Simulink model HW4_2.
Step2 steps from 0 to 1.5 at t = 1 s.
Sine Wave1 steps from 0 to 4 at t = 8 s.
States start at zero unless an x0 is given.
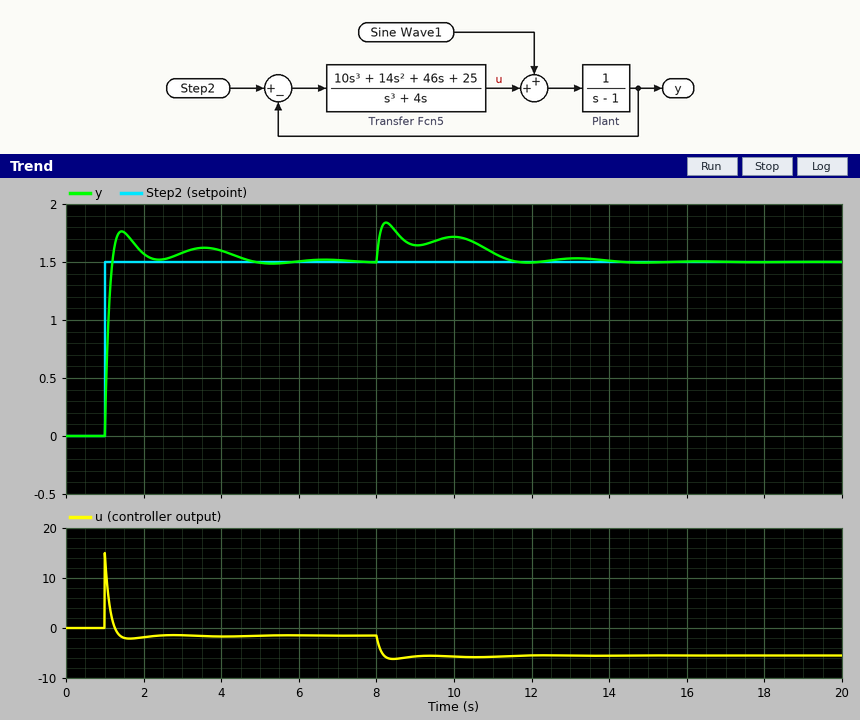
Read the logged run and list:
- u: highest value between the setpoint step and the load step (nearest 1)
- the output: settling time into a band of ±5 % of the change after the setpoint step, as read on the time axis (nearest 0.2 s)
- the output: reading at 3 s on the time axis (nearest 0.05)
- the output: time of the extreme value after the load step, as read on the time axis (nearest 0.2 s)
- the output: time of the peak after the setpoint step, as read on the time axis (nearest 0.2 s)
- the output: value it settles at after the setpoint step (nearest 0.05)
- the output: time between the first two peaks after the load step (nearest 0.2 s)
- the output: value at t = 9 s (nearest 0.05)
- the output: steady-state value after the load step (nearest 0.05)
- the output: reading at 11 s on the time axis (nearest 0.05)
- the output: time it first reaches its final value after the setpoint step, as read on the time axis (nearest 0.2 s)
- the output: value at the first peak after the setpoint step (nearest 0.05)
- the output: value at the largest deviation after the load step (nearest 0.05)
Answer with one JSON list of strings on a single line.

["15", "4.2 s", "1.60", "8.2 s", "1.4 s", "1.50", "1.8 s", "1.65", "1.50", "1.60", "1.2 s", "1.75", "1.85"]
